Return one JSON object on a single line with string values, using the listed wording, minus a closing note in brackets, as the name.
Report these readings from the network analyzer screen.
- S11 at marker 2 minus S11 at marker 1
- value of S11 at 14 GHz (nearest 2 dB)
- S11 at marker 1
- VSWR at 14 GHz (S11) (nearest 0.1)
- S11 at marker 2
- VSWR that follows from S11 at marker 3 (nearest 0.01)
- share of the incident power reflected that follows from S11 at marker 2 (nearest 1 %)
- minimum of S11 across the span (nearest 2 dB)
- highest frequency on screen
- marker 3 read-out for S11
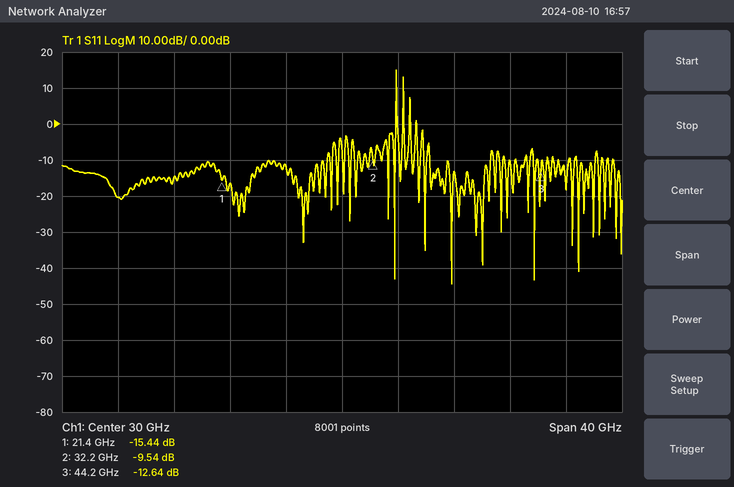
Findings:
{"S11 at marker 2 minus S11 at marker 1": "5.90 dB", "value of S11 at 14 GHz": "-20 dB", "S11 at marker 1": "-15.44 dB", "VSWR at 14 GHz (S11)": "1.2", "S11 at marker 2": "-9.54 dB", "VSWR that follows from S11 at marker 3": "1.61", "share of the incident power reflected that follows from S11 at marker 2": "11 %", "minimum of S11 across the span": "-44 dB", "highest frequency on screen": "50 GHz", "marker 3 read-out for S11": "-12.64 dB"}
